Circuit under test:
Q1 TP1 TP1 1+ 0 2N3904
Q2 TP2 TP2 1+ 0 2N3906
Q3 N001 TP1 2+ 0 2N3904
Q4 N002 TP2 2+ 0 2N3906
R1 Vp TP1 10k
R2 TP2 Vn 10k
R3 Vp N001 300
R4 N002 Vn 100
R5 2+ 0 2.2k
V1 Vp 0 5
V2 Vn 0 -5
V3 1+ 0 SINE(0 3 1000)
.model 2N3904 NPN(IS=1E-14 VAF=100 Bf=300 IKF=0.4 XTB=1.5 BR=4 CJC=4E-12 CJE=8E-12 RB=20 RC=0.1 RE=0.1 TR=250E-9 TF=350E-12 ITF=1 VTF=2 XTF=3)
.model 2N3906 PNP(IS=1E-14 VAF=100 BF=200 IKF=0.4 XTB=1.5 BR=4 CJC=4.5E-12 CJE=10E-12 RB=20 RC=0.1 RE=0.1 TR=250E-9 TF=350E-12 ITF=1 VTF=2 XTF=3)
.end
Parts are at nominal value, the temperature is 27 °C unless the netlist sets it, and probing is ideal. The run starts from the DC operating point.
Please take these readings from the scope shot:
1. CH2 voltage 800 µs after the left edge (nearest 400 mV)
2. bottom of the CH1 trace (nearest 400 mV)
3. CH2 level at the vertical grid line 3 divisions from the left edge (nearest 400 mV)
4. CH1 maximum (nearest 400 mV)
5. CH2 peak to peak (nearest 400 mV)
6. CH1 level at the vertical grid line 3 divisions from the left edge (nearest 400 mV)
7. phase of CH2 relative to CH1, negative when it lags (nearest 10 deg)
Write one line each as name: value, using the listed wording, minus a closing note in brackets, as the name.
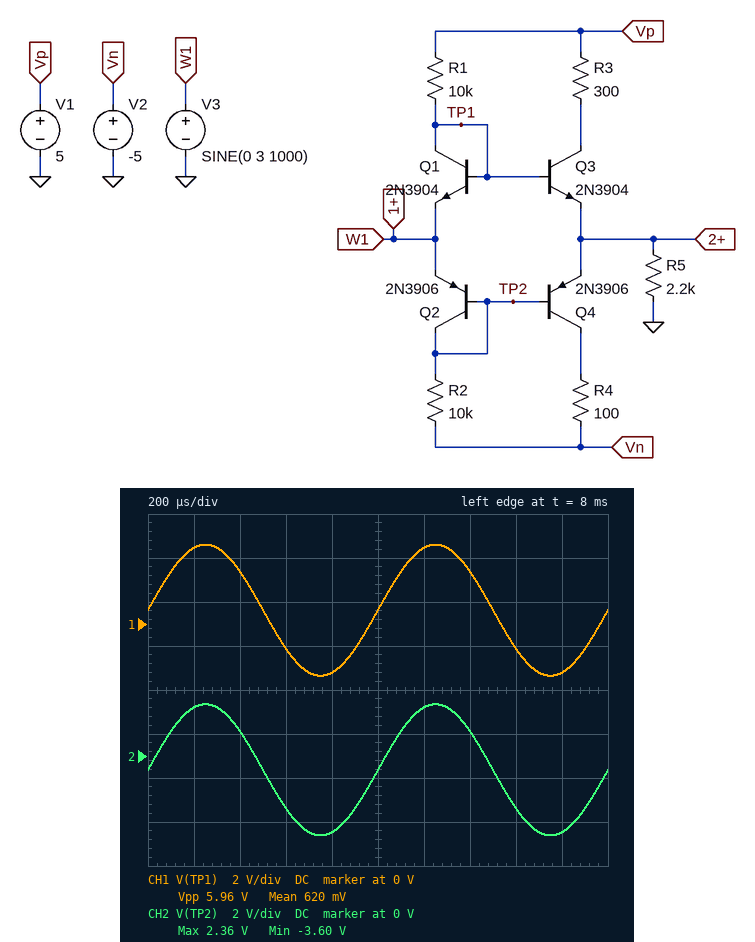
CH2 voltage 800 µs after the left edge: -3.6 V
bottom of the CH1 trace: -2.4 V
CH2 level at the vertical grid line 3 divisions from the left edge: -2.4 V
CH1 maximum: 3.6 V
CH2 peak to peak: 6.0 V
CH1 level at the vertical grid line 3 divisions from the left edge: -1.2 V
phase of CH2 relative to CH1, negative when it lags: 0 deg
